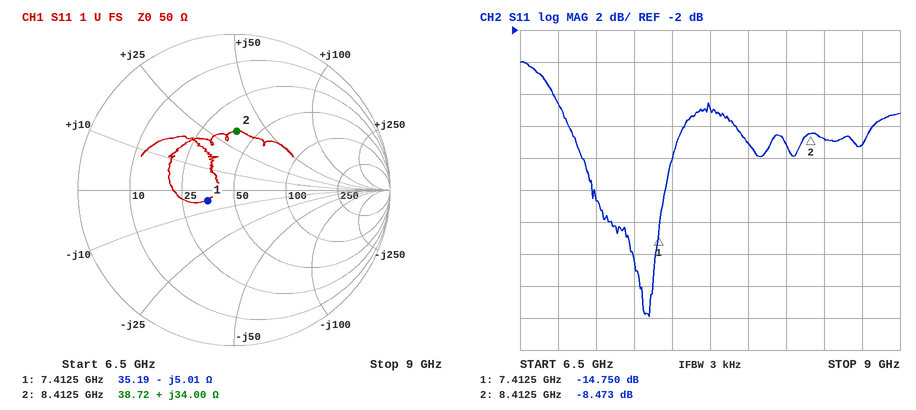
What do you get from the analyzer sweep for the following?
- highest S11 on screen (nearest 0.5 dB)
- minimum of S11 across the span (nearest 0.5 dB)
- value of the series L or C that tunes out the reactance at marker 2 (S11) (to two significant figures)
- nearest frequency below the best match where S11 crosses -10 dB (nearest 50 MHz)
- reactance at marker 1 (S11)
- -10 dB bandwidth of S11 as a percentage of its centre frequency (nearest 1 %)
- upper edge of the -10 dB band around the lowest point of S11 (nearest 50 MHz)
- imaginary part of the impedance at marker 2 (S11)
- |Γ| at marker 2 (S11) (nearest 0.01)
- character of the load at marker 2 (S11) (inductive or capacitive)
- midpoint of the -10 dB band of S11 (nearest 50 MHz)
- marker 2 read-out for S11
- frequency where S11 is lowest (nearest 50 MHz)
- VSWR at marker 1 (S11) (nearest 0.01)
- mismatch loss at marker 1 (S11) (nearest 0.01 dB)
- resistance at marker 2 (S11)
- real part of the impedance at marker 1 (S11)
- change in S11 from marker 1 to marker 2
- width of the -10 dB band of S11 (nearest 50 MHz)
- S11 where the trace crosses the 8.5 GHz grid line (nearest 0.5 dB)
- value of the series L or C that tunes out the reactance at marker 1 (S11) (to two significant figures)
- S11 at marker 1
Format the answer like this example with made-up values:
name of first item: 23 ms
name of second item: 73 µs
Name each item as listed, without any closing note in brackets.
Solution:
highest S11 on screen: -4.0 dB
minimum of S11 across the span: -20.0 dB
value of the series L or C that tunes out the reactance at marker 2 (S11): 560 fF
nearest frequency below the best match where S11 crosses -10 dB: 6.90 GHz
reactance at marker 1: -5.01 Ω
-10 dB bandwidth of S11 as a percentage of its centre frequency: 8 %
upper edge of the -10 dB band around the lowest point of S11: 7.50 GHz
imaginary part of the impedance at marker 2: +34.00 Ω
|Γ| at marker 2 (S11): 0.38
character of the load at marker 2 (S11): inductive
midpoint of the -10 dB band of S11: 7.20 GHz
marker 2 read-out for S11: -8.473 dB
frequency where S11 is lowest: 7.35 GHz
VSWR at marker 1 (S11): 1.45
mismatch loss at marker 1 (S11): 0.15 dB
resistance at marker 2: 38.72 Ω
real part of the impedance at marker 1: 35.19 Ω
change in S11 from marker 1 to marker 2: 6.277 dB
width of the -10 dB band of S11: 600 MHz
S11 where the trace crosses the 8.5 GHz grid line: -9.0 dB
value of the series L or C that tunes out the reactance at marker 1 (S11): 110 pH
S11 at marker 1: -14.750 dB
